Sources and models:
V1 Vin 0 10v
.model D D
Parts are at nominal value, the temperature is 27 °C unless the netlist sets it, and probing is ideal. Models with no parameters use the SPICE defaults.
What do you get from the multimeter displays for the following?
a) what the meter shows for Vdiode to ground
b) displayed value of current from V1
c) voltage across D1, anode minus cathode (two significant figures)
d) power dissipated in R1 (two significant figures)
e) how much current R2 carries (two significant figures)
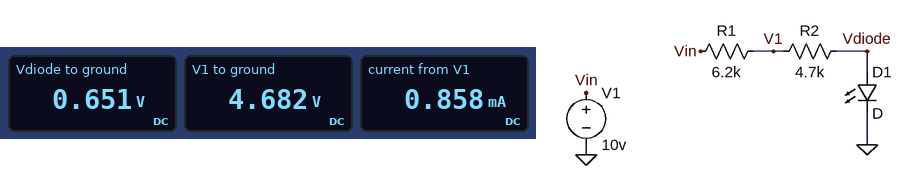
0.651 V
0.858 mA
650 mV
4.6 mW
860 µA
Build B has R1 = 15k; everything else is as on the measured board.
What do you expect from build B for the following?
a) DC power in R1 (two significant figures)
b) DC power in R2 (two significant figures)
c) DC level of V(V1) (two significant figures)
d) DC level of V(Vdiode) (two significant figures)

3.4 mW
1.1 mW
2.9 V
640 mV
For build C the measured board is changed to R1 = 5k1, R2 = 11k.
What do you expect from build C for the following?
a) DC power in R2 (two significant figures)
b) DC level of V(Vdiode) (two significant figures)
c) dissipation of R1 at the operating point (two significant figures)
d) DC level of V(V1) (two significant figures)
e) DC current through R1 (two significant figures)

3.7 mW
640 mV
1.7 mW
7.0 V
580 µA
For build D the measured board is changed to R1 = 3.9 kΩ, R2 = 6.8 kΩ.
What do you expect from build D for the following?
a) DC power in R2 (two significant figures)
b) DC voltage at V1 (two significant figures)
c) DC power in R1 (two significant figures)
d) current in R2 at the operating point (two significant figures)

5.2 mW
6.6 V
3.0 mW
870 µA
